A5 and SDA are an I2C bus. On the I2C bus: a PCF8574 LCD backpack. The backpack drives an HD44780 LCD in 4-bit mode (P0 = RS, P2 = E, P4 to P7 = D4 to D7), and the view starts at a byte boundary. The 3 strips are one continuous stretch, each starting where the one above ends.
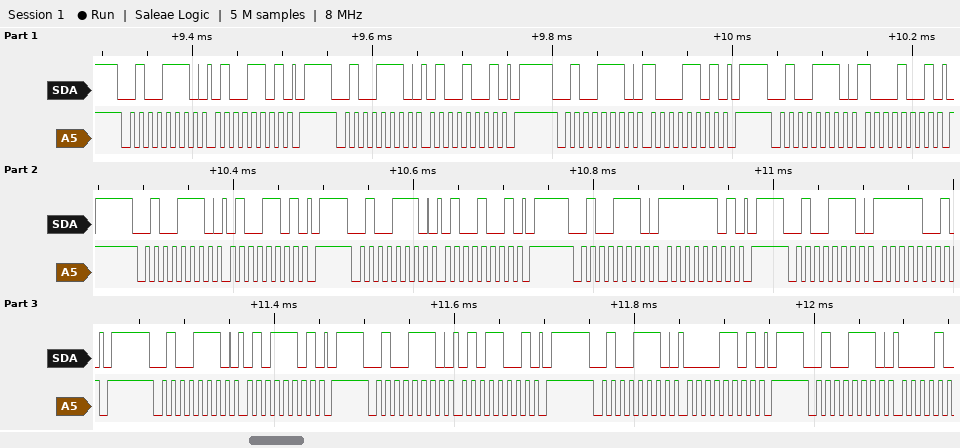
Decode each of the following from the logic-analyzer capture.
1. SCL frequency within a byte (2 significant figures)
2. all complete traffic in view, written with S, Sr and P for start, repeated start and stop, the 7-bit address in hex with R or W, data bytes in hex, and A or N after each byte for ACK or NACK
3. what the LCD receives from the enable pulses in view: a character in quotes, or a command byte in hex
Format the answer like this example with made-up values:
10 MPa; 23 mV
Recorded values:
100 kHz; S 27W A 4D A P S 27W A 49 A P S 27W A 8D A P S 27W A 89 A P S 27W A 4D A P S 27W A 49 A P S 27W A FD A P S 27W A F9 A P S 27W A 5D A P S 27W A 59 A P S 27W A 0D A P S 27W A; 'H' 'O'
